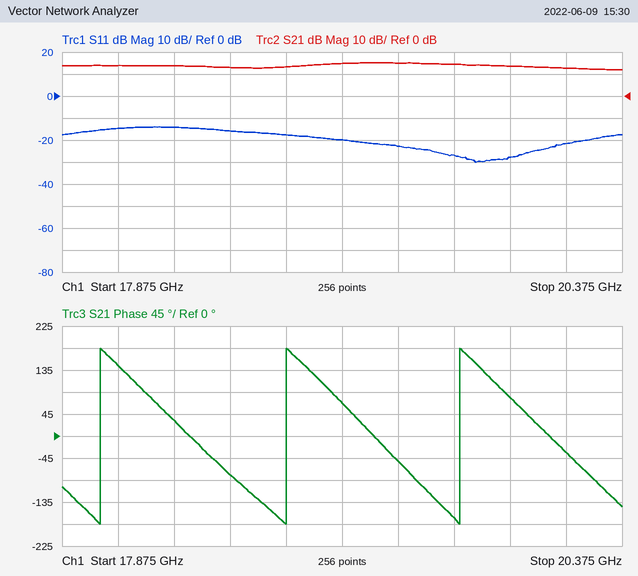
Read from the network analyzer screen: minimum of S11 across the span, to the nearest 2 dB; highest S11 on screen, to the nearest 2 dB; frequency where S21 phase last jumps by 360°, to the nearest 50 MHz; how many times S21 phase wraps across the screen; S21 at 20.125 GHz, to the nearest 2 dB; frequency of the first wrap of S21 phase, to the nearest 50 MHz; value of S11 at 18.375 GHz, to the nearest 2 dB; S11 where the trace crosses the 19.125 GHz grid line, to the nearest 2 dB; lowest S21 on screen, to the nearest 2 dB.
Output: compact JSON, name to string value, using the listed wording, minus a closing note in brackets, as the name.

{"minimum of S11 across the span, to the nearest 2 dB": "-30 dB", "highest S11 on screen, to the nearest 2 dB": "-14 dB", "frequency where S21 phase last jumps by 360°, to the nearest 50 MHz": "19.65 GHz", "how many times S21 phase wraps across the screen": "3", "S21 at 20.125 GHz, to the nearest 2 dB": "12 dB", "frequency of the first wrap of S21 phase, to the nearest 50 MHz": "18.05 GHz", "value of S11 at 18.375 GHz, to the nearest 2 dB": "-14 dB", "S11 where the trace crosses the 19.125 GHz grid line, to the nearest 2 dB": "-20 dB", "lowest S21 on screen, to the nearest 2 dB": "12 dB"}
